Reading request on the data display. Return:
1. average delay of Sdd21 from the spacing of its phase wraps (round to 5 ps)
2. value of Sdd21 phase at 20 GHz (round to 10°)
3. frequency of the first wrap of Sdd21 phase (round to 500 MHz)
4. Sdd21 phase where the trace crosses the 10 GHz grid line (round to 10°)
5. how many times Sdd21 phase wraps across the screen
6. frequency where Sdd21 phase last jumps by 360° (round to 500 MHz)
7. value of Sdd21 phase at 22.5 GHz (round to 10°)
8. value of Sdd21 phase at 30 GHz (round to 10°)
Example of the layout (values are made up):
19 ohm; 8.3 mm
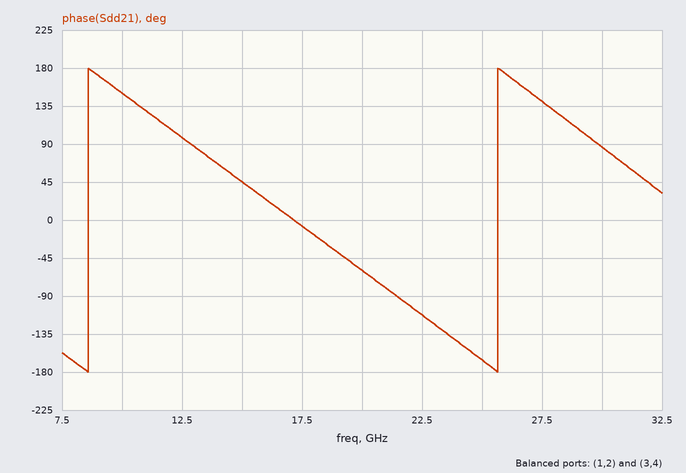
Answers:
60 ps; -60°; 8.5 GHz; 150°; 2; 25.5 GHz; -110°; 90°
